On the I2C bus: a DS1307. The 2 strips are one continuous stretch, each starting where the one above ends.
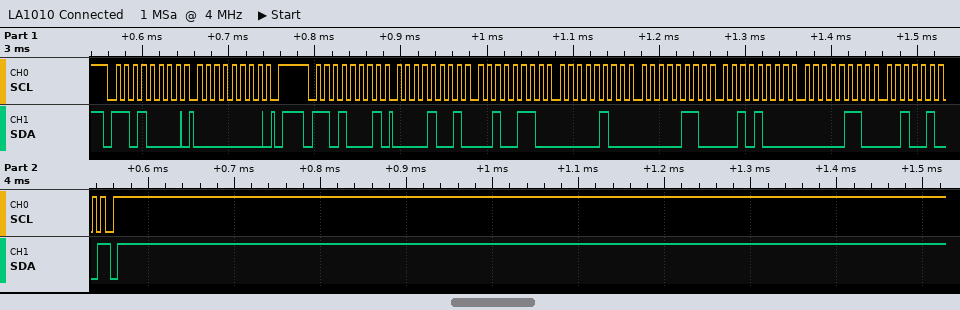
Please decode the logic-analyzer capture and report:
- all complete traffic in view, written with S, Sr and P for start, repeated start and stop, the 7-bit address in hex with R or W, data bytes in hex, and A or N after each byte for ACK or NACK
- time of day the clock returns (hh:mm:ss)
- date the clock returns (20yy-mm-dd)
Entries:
S 68W A 00 A P S 68R A 09 A 26 A 04 A 06 A 28 A 06 A 24 N P
04:26:09
2024-06-28
